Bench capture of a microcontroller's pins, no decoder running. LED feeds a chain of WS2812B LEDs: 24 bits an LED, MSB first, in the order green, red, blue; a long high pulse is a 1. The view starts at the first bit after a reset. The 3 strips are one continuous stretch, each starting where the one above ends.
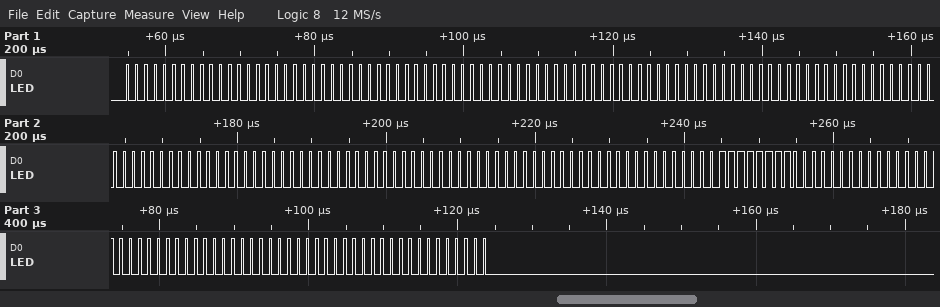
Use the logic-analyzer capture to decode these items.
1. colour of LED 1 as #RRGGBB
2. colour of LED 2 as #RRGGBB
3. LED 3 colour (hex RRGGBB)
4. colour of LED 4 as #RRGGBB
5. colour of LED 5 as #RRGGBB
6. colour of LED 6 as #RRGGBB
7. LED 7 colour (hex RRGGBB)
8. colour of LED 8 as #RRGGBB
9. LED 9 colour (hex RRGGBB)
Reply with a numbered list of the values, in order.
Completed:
1. #000000
2. #000000
3. #000000
4. #000000
5. #000000
6. #000000
7. #FF0000
8. #000000
9. #000000
